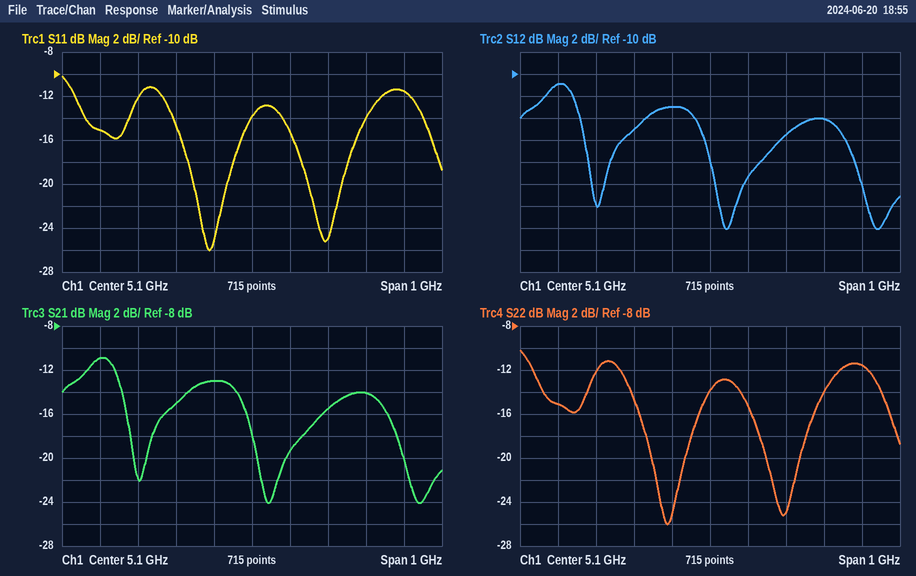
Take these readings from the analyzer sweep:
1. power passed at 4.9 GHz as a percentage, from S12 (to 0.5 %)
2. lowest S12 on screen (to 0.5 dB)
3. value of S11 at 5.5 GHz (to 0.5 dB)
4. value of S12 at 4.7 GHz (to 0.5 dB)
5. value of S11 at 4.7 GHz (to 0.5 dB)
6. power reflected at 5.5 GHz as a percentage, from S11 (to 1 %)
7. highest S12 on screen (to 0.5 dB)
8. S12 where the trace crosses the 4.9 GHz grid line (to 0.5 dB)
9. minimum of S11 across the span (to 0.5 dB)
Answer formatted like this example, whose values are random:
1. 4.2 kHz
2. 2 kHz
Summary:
1. 3.0 %
2. -24.0 dB
3. -11.5 dB
4. -11.0 dB
5. -15.0 dB
6. 7 %
7. -11.0 dB
8. -15.0 dB
9. -26.0 dB
